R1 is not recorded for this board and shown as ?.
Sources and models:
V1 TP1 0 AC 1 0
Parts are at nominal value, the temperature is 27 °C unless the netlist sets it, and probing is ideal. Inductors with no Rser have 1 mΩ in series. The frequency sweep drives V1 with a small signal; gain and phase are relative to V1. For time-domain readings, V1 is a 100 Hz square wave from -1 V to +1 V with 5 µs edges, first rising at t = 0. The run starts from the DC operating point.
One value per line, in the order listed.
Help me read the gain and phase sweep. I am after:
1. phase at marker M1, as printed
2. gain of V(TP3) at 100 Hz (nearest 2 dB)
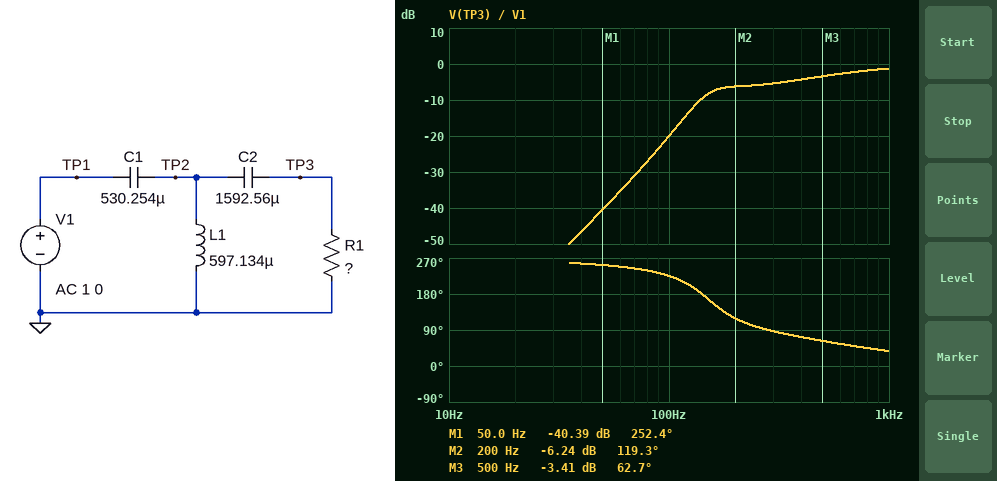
252.4 deg
-20 dB
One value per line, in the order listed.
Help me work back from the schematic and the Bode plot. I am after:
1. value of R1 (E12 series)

0.56 Ω
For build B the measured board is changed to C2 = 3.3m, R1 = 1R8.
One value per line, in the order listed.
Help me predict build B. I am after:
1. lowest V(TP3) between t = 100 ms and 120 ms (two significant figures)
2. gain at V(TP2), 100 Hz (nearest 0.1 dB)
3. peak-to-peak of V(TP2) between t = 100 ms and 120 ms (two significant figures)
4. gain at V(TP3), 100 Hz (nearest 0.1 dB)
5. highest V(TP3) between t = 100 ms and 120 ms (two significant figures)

-2.1 V
-16.6 dB
4.2 V
-16.9 dB
2.1 V
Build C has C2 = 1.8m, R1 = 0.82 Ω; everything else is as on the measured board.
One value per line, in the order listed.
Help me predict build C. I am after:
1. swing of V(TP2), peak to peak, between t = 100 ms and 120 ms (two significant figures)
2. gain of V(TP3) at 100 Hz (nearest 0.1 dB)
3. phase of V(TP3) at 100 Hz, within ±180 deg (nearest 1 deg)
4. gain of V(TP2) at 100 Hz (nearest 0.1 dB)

3.8 V
-18.1 dB
-151 deg
-14.7 dB
